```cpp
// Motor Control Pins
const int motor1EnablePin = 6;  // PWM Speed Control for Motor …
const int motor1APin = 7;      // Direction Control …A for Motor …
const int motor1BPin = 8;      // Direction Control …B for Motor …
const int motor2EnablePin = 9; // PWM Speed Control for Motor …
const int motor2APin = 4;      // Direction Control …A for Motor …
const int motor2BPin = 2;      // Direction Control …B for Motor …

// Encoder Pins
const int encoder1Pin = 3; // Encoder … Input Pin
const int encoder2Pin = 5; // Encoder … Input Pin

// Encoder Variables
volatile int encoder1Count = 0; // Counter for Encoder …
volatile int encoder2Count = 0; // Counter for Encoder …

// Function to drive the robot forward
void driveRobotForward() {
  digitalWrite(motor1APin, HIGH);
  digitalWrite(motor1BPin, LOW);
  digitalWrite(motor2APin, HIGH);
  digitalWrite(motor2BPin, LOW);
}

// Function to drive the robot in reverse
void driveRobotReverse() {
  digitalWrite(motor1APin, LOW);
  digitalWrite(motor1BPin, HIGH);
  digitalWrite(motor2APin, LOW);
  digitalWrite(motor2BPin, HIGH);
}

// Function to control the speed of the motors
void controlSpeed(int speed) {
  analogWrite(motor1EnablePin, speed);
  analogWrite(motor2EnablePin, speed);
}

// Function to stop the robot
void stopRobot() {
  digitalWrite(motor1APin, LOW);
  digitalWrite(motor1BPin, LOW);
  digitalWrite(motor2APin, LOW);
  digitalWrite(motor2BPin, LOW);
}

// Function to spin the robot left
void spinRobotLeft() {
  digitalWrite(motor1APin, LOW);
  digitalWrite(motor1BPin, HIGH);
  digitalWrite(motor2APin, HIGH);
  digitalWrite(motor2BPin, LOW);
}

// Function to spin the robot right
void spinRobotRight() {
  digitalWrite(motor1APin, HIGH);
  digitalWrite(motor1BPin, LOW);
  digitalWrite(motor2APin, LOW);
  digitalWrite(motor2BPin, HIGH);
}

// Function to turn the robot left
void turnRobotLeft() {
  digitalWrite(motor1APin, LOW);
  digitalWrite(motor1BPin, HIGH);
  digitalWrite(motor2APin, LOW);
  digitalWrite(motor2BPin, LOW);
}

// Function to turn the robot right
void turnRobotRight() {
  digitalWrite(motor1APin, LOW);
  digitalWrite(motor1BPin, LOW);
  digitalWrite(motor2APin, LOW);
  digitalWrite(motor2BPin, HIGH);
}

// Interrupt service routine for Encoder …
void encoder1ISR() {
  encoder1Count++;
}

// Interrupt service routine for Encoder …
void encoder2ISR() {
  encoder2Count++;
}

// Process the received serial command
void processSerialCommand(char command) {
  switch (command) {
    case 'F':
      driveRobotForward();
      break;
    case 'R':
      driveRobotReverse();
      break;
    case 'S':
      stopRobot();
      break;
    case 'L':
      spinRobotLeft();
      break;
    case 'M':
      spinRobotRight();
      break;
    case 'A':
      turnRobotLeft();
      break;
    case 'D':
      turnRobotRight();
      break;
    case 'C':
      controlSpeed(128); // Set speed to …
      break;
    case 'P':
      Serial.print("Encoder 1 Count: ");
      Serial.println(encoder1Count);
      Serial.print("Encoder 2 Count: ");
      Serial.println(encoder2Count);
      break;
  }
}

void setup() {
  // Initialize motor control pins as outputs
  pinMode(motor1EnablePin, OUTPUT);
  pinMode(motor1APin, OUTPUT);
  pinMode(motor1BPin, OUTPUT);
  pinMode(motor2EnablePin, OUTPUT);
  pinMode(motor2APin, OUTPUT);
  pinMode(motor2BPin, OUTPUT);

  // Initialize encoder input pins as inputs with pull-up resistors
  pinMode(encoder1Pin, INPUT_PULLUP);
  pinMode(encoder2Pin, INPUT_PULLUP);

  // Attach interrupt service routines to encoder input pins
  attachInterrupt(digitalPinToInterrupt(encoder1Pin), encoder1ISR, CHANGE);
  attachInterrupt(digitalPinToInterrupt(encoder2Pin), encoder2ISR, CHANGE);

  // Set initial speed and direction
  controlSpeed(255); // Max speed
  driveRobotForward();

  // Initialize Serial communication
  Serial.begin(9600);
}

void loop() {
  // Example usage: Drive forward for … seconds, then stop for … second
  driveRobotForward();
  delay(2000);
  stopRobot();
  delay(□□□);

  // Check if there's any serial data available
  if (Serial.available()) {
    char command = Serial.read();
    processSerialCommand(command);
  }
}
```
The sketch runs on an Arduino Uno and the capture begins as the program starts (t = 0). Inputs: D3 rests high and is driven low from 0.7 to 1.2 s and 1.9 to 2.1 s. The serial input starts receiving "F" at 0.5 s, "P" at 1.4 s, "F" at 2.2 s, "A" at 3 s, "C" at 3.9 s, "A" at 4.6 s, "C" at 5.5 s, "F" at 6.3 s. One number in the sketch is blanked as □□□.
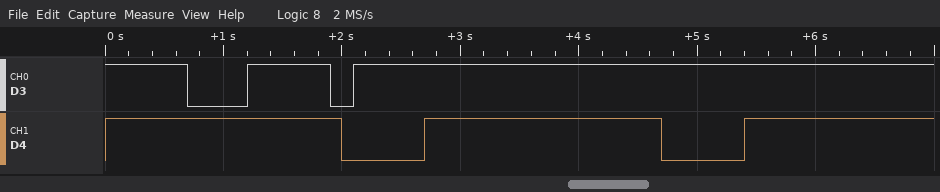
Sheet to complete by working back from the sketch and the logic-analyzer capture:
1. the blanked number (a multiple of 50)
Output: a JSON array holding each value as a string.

["700"]
